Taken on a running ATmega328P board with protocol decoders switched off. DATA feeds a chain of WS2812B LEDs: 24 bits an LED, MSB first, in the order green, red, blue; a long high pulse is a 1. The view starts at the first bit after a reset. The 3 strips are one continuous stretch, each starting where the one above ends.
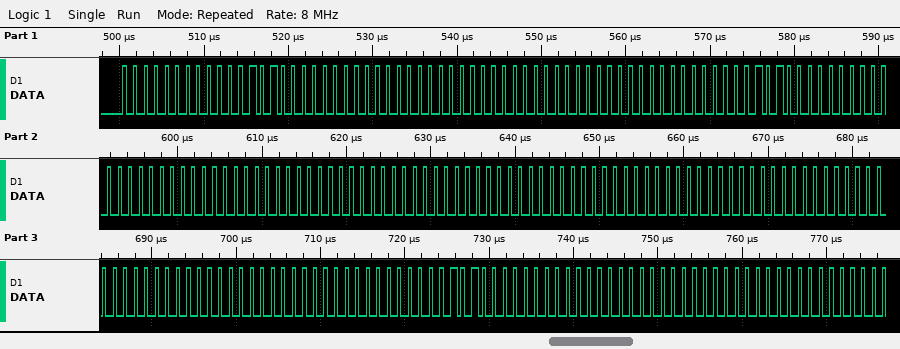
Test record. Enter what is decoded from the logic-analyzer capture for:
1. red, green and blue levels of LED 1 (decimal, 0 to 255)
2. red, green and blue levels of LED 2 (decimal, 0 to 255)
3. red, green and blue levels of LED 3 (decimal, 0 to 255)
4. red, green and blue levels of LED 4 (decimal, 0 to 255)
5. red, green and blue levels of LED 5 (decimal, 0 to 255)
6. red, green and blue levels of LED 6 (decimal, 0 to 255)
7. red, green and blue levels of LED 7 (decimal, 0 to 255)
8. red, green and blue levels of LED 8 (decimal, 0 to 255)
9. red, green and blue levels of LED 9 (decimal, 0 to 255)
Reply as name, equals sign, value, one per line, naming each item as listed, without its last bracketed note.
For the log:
red, green and blue levels of LED 1 = 10, 0, 0
red, green and blue levels of LED 2 = 0, 0, 0
red, green and blue levels of LED 3 = 10, 0, 0
red, green and blue levels of LED 4 = 0, 0, 0
red, green and blue levels of LED 5 = 0, 0, 0
red, green and blue levels of LED 6 = 0, 0, 0
red, green and blue levels of LED 7 = 0, 0, 0
red, green and blue levels of LED 8 = 10, 0, 0
red, green and blue levels of LED 9 = 0, 0, 0
